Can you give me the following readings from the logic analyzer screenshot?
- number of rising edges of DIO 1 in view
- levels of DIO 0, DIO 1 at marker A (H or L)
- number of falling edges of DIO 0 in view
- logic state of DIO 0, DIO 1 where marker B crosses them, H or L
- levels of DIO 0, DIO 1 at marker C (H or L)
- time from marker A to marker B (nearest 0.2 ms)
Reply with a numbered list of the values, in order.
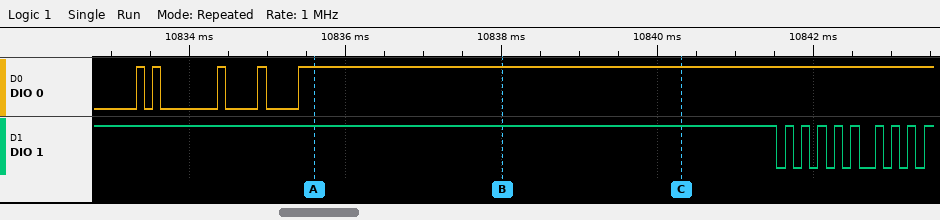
1. 9
2. DIO 0=H, DIO 1=H
3. 4
4. DIO 0=H, DIO 1=H
5. DIO 0=H, DIO 1=H
6. 2.4 ms
